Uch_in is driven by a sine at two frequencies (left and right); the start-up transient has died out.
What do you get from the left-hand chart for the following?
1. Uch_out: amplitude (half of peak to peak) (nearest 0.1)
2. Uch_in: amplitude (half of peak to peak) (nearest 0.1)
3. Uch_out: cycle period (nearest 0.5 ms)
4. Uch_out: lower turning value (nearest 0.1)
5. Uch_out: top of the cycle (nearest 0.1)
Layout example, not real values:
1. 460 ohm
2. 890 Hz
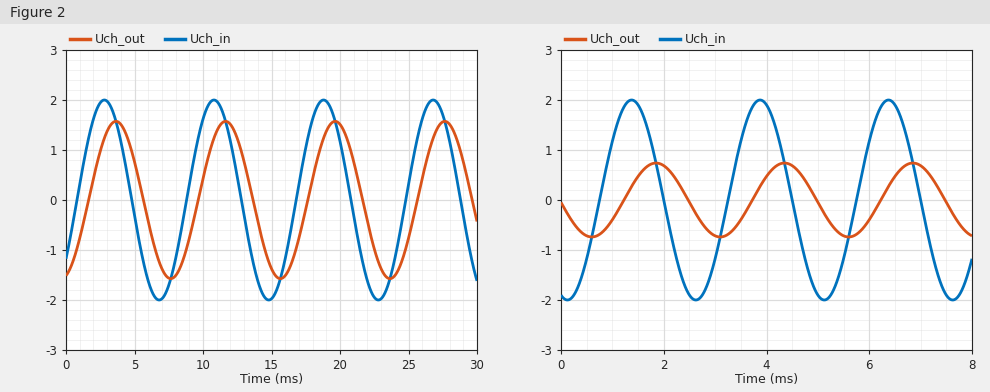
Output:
1. 1.6
2. 2.0
3. 8.0 ms
4. -1.6
5. 1.6
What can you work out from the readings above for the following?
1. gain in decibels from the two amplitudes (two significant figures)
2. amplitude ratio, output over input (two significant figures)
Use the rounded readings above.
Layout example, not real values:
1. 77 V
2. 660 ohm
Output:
1. -1.9 dB
2. 0.80
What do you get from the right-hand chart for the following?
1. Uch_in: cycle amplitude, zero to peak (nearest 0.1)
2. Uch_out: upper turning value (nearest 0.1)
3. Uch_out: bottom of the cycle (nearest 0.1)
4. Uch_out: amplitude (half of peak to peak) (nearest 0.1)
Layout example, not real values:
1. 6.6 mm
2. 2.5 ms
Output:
1. 2.0
2. 0.7
3. -0.7
4. 0.7
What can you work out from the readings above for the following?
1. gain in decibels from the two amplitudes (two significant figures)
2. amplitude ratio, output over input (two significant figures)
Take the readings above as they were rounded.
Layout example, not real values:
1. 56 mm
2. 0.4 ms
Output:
1. -9.1 dB
2. 0.35
